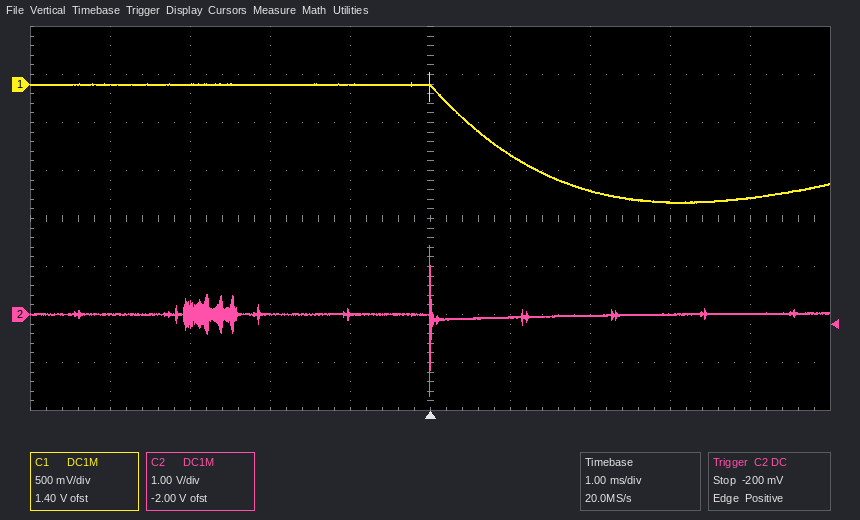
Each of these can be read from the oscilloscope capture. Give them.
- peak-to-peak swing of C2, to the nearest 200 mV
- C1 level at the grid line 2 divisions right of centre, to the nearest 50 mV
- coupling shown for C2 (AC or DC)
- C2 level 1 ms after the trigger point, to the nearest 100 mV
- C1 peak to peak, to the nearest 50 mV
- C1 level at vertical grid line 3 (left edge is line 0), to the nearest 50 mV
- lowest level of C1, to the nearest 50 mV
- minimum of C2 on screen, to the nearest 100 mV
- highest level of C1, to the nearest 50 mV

3.2 V
-1.10 V
DC
-100 mV
1.35 V
0 mV
-1.25 V
-1.7 V
100 mV
